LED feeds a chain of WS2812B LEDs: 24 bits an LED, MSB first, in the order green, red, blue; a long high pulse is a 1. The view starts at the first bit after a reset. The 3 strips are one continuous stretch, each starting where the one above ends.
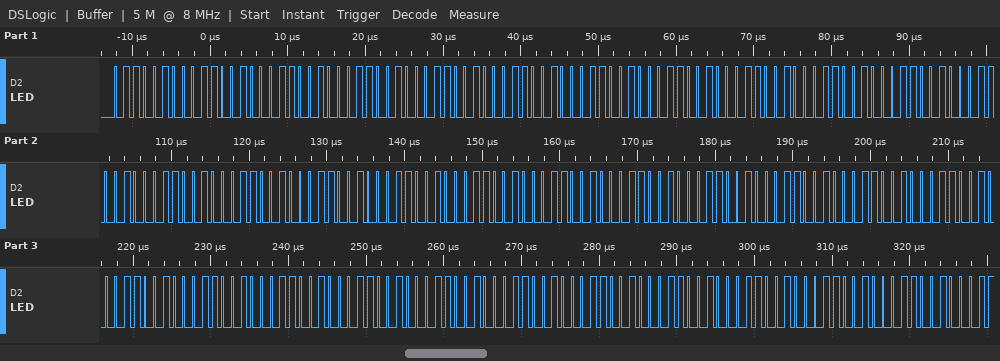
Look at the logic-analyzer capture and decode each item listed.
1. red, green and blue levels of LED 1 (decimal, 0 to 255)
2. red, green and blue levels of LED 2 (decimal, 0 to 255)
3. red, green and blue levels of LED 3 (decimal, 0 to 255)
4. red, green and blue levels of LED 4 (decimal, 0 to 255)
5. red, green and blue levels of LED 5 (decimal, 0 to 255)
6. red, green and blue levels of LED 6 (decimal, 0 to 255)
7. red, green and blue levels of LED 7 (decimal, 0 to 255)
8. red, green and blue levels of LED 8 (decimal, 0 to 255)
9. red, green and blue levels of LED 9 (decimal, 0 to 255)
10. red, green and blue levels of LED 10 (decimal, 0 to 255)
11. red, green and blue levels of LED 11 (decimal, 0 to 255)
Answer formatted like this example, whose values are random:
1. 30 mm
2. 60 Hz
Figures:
1. 100, 100, 100
2. 100, 100, 100
3. 100, 100, 100
4. 100, 100, 100
5. 100, 100, 100
6. 100, 100, 100
7. 100, 100, 100
8. 100, 100, 100
9. 100, 100, 100
10. 100, 100, 100
11. 100, 100, 100
